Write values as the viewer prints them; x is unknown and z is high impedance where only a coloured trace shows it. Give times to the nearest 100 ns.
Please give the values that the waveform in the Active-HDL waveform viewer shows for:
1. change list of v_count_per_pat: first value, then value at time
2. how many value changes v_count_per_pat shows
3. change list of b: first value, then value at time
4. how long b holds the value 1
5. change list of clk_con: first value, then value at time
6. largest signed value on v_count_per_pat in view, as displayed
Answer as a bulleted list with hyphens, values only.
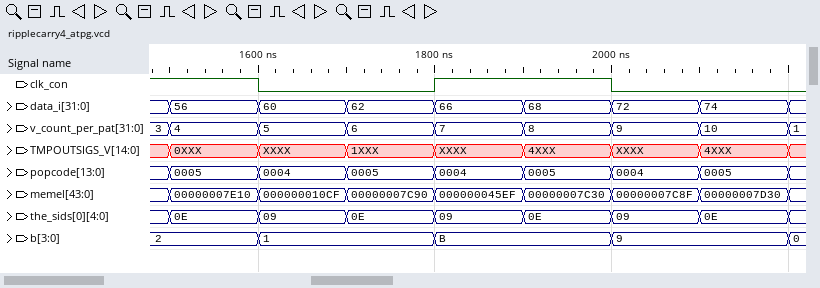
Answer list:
- 3, 4 at 1500 ns, 5 at 1600 ns, 6 at 1700 ns, 7 at 1800 ns, 8 at 1900 ns, 9 at 2000 ns, 10 at 2100 ns, 1 at 2200 ns
- 8
- 2, 1 at 1600 ns, B at 1800 ns, 9 at 2000 ns, 0 at 2200 ns
- 200 ns
- 1, 0 at 1600 ns, 1 at 1800 ns, 0 at 2000 ns
- 10
